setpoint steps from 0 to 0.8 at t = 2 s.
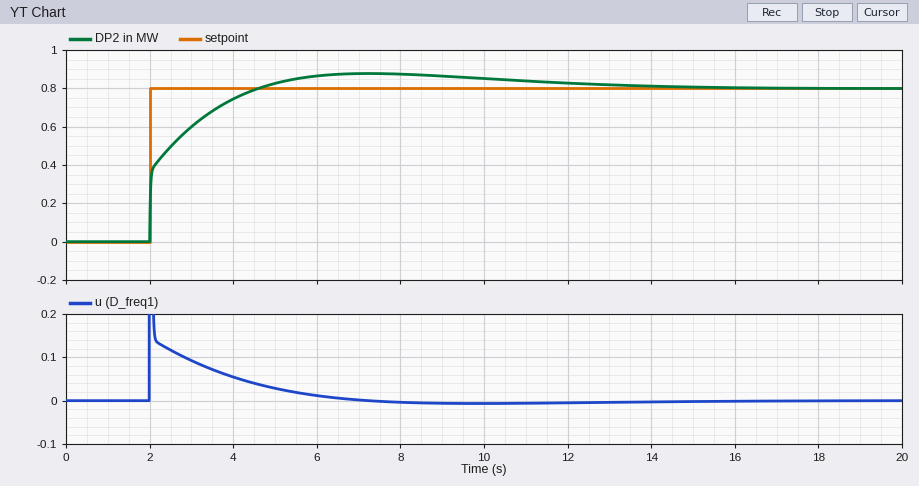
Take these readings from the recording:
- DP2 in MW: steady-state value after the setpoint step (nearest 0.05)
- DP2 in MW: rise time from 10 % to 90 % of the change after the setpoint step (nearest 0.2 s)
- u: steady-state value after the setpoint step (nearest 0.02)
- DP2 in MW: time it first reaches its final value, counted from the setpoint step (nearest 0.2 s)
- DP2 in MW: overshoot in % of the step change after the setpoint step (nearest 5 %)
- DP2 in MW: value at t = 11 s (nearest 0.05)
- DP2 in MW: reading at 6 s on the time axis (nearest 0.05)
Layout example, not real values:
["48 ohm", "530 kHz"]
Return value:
["0.80", "1.8 s", "0.00", "2.6 s", "10 %", "0.85", "0.85"]
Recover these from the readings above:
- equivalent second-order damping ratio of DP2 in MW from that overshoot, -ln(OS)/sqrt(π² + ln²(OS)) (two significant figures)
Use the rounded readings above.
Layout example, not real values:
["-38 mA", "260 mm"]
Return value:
["0.59"]
